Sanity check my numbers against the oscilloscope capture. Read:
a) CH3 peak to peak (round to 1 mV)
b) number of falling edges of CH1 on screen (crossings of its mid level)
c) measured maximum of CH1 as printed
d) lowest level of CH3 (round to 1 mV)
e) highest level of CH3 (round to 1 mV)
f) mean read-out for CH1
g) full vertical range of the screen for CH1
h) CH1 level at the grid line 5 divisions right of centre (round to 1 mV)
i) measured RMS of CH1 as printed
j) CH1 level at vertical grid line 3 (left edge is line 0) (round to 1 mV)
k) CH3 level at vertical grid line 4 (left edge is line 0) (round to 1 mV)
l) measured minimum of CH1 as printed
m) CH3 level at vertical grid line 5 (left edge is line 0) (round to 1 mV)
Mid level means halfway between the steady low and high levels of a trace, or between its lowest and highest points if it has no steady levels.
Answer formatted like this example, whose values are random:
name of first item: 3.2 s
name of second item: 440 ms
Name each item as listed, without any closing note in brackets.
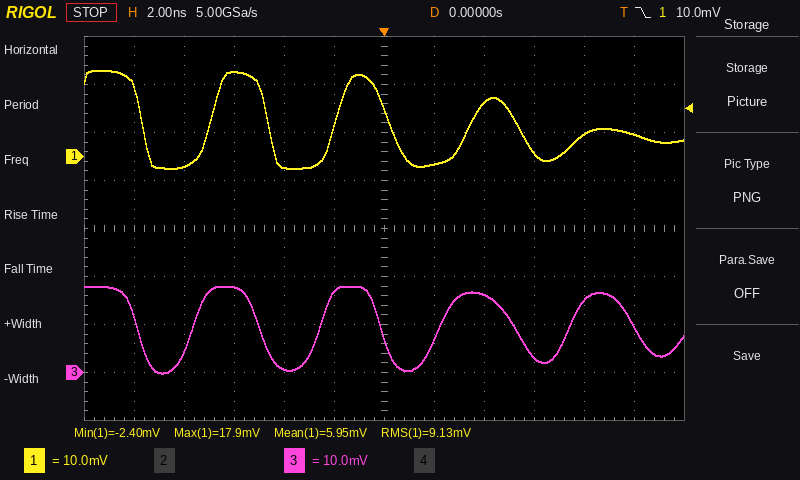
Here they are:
CH3 peak to peak: 18 mV
number of falling edges of CH1 on screen: 4
measured maximum of CH1 as printed: 17.9 mV
lowest level of CH3: 0 mV
highest level of CH3: 18 mV
mean read-out for CH1: 5.95 mV
full vertical range of the screen for CH1: 80 mV
CH1 level at the grid line 5 divisions right of centre: 5 mV
measured RMS of CH1 as printed: 9.13 mV
CH1 level at vertical grid line 3 (left edge is line 0): 18 mV
CH3 level at vertical grid line 4 (left edge is line 0): 1 mV
measured minimum of CH1 as printed: -2.40 mV
CH3 level at vertical grid line 5 (left edge is line 0): 17 mV
